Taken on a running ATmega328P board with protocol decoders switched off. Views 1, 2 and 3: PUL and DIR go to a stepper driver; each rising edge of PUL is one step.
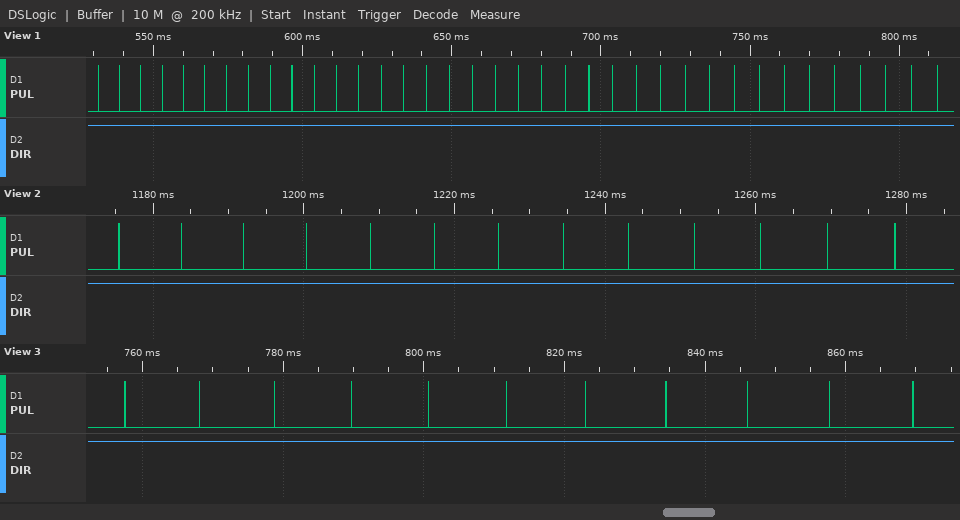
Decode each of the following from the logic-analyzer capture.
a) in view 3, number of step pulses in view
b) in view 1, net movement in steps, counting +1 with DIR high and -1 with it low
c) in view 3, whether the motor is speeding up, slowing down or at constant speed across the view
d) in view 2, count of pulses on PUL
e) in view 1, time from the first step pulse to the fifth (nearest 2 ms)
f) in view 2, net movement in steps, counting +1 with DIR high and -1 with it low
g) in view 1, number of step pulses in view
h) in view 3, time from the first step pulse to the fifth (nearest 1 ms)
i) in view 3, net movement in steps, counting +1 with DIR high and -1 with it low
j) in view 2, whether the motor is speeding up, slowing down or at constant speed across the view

11
+37
slowing down
13
28 ms
+13
37
43 ms
+11
slowing down
